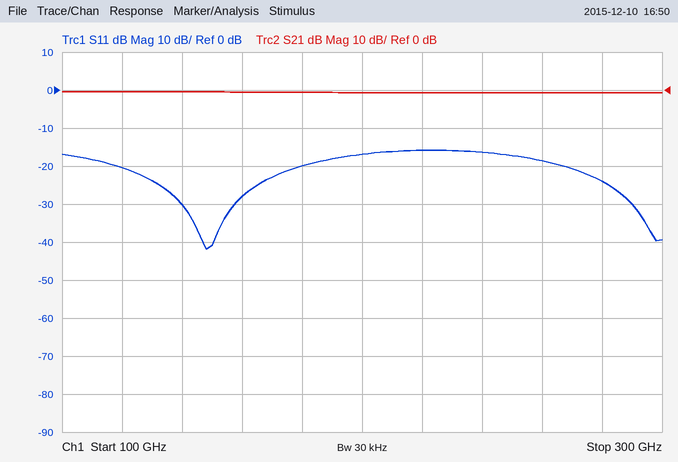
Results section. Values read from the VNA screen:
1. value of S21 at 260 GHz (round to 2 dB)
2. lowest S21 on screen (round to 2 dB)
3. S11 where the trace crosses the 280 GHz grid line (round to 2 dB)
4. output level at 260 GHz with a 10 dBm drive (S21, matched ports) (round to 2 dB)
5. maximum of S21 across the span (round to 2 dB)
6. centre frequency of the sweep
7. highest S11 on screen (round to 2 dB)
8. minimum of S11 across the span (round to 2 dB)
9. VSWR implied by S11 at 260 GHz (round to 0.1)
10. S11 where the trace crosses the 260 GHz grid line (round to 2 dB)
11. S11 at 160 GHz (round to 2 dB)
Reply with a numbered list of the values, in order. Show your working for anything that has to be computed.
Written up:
1. 0 dB
2. 0 dB
3. -24 dB
4. 10 dBm + (0 dB) = 10 dBm
5. 0 dB
6. 200 GHz
7. -16 dB
8. -42 dB
9. |Γ| = 10^(-18/20) = 0.1259; VSWR = (1 + 0.1259)/(1 − 0.1259) ≈ 1.3
10. -18 dB
11. -28 dB
